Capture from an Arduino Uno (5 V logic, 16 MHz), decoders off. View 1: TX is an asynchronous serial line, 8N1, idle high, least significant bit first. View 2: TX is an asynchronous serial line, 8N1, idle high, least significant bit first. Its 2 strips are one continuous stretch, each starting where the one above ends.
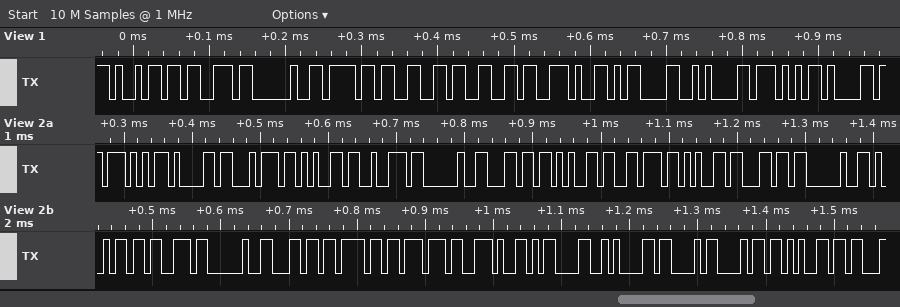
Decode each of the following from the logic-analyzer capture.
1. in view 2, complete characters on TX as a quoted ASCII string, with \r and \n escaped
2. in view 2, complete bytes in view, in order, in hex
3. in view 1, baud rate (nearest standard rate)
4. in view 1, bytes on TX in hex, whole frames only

"Water level is low.\r\nChe"
57 61 74 65 72 20 6C 65 76 65 6C 20 69 73 20 6C 6F 77 2E 0D 0A 43 68 65
115200 baud
69 73 20 6F 66 66 2E 0D 0A 57 61
